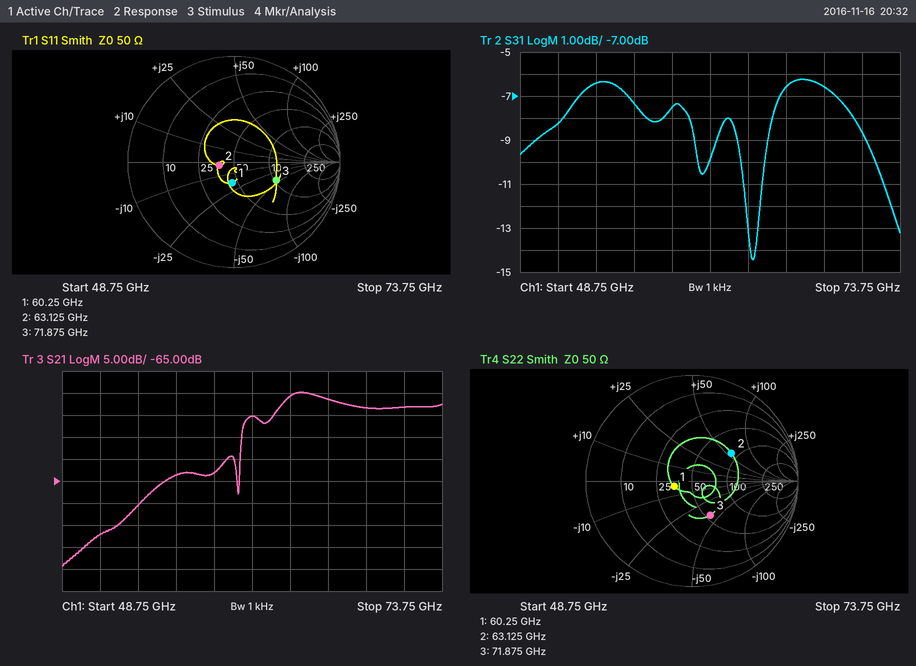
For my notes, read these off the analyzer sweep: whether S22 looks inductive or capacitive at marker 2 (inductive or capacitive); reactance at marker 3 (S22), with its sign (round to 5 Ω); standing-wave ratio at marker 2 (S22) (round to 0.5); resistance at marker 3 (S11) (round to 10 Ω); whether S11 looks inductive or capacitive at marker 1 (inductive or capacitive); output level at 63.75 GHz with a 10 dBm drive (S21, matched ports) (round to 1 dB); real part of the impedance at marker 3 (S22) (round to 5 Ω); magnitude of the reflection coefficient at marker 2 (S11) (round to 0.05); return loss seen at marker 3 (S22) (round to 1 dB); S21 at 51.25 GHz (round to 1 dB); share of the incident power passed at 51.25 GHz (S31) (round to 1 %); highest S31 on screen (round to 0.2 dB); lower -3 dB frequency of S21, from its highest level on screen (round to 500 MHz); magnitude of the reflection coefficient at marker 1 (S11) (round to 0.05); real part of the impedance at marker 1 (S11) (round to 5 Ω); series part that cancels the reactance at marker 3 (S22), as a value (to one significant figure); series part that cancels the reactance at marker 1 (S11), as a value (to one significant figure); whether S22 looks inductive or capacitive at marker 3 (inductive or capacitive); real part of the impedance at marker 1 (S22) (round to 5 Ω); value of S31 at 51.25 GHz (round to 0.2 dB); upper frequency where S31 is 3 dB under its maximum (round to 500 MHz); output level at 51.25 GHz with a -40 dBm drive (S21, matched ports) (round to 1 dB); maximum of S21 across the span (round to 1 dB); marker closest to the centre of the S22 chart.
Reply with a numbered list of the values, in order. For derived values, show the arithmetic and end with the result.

1. inductive
2. -40 Ω
3. 2.5
4. 100 Ω
5. capacitive
6. 10 dBm + (-46 dB) = -36 dBm
7. 55 Ω
8. 0.15
9. 9 dB
10. -77 dB
11. 10^(-8.2/10) ≈ 15 %
12. -6.2 dB
13. 63.0 GHz
14. 0.20
15. 45 Ω
16. L = 40 Ω/(2π × 71.875 GHz) ≈ 88.6 pH, so 90 pH to one significant figure
17. L = 20 Ω/(2π × 60.25 GHz) ≈ 52.8 pH, so 50 pH to one significant figure
18. capacitive
19. 35 Ω
20. -8.2 dB
21. 71.5 GHz
22. -40 dBm + (-77 dB) = -117 dBm
23. -45 dB
24. marker 1
